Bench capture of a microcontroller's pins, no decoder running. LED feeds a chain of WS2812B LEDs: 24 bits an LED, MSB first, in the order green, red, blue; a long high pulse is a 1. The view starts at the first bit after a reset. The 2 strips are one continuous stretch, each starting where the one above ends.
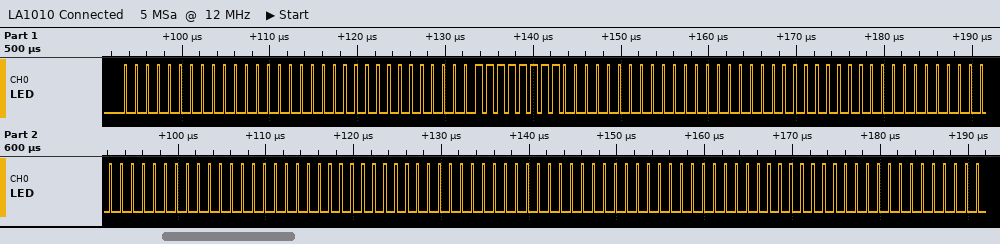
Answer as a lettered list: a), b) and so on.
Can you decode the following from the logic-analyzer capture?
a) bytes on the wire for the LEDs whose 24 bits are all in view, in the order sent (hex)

a) 00 00 00 00 FF 00 00 00 00 00 00 00 00 00 00 00 00 00
